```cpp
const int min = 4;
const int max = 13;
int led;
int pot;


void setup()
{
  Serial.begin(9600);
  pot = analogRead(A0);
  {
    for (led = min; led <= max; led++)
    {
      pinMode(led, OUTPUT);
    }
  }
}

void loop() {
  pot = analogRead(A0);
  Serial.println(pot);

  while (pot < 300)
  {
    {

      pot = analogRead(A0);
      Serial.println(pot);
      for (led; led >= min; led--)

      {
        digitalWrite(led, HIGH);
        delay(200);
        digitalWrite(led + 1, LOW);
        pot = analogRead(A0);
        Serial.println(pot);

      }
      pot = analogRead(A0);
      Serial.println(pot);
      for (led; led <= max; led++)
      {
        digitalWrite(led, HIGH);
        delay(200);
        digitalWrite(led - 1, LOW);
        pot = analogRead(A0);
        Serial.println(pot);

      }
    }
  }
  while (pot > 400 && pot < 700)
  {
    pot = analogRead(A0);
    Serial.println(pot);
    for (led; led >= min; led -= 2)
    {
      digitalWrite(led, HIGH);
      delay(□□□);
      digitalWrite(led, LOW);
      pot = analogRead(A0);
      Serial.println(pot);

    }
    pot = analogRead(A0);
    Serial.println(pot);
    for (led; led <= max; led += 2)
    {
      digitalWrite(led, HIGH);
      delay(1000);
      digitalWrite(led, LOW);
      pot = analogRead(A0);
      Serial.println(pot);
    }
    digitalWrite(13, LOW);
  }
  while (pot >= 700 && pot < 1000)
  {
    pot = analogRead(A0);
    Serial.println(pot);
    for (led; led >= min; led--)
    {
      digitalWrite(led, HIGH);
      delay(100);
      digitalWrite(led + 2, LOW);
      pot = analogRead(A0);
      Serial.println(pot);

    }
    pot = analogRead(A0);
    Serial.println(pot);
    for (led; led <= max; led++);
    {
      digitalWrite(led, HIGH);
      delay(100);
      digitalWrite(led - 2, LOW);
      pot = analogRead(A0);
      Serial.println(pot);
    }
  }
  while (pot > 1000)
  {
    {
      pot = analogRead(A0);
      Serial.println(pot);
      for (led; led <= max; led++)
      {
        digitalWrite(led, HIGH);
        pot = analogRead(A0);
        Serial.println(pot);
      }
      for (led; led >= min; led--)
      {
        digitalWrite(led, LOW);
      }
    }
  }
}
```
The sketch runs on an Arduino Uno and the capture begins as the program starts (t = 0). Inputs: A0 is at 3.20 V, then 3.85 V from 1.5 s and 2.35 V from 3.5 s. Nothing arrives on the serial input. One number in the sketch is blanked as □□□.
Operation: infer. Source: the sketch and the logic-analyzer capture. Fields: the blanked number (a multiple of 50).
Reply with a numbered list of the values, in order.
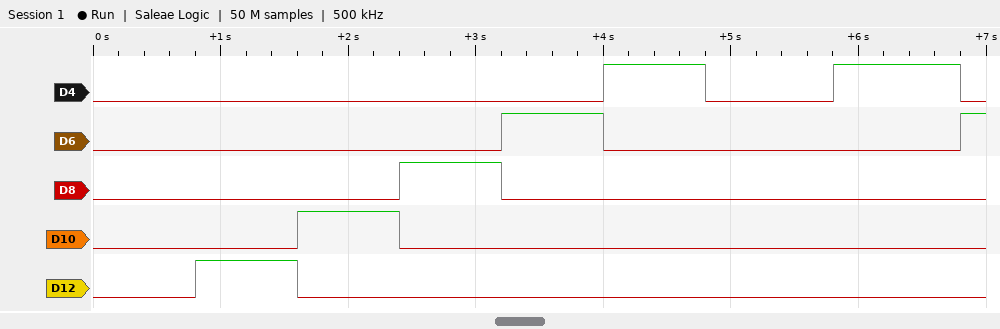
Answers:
1. 800
